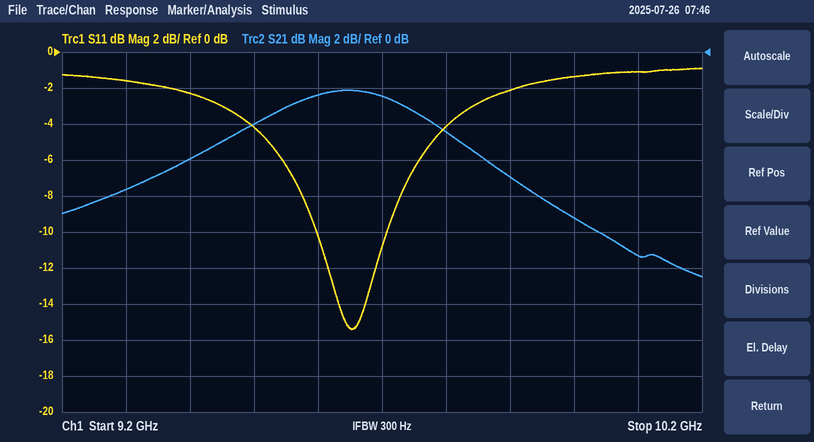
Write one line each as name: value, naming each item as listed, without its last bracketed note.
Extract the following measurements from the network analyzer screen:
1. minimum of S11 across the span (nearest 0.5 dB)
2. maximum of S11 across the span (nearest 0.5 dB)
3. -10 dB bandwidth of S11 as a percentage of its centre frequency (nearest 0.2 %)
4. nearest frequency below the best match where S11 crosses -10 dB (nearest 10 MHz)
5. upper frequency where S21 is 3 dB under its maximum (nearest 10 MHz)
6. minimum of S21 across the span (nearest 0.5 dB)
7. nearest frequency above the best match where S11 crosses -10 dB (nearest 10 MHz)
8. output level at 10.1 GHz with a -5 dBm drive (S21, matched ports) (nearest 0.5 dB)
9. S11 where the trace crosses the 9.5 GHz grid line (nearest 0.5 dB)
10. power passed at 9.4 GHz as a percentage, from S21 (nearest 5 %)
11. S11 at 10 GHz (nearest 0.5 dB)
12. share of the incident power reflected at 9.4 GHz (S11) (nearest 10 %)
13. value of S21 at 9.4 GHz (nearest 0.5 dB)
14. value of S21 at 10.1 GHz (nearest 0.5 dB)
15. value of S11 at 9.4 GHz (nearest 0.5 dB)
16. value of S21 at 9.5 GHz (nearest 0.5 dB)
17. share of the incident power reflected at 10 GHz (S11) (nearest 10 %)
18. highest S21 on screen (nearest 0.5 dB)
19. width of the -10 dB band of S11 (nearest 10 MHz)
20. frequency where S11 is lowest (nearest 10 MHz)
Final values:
minimum of S11 across the span: -15.5 dB
maximum of S11 across the span: -1.0 dB
-10 dB bandwidth of S11 as a percentage of its centre frequency: 1.2 %
nearest frequency below the best match where S11 crosses -10 dB: 9.60 GHz
upper frequency where S21 is 3 dB under its maximum: 9.83 GHz
minimum of S21 across the span: -12.5 dB
nearest frequency above the best match where S11 crosses -10 dB: 9.71 GHz
output level at 10.1 GHz with a -5 dBm drive (S21, matched ports): -16.5 dBm
S11 where the trace crosses the 9.5 GHz grid line: -4.0 dB
power passed at 9.4 GHz as a percentage, from S21: 25 %
S11 at 10 GHz: -1.5 dB
share of the incident power reflected at 9.4 GHz (S11): 60 %
value of S21 at 9.4 GHz: -6.0 dB
value of S21 at 10.1 GHz: -11.5 dB
value of S11 at 9.4 GHz: -2.5 dB
value of S21 at 9.5 GHz: -4.0 dB
share of the incident power reflected at 10 GHz (S11): 70 %
highest S21 on screen: -2.0 dB
width of the -10 dB band of S11: 110 MHz
frequency where S11 is lowest: 9.65 GHz
